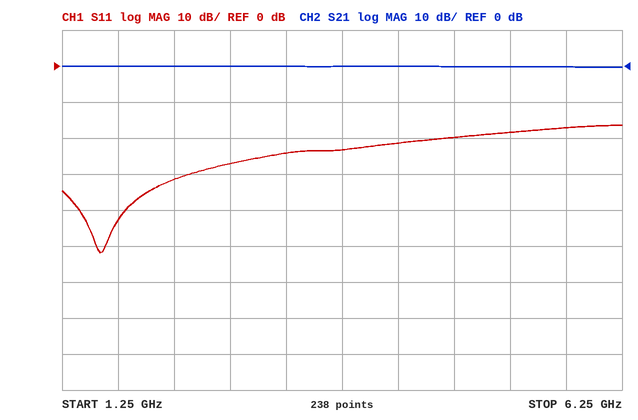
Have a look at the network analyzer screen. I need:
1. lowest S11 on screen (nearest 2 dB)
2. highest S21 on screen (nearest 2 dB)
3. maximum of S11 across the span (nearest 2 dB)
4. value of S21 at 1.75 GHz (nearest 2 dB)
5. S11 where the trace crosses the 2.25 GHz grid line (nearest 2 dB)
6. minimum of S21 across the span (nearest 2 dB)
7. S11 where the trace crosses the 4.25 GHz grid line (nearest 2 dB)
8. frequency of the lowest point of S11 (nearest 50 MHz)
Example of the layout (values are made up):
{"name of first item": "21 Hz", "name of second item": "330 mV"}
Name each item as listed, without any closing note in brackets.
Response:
{"lowest S11 on screen": "-52 dB", "highest S21 on screen": "0 dB", "maximum of S11 across the span": "-16 dB", "value of S21 at 1.75 GHz": "0 dB", "S11 where the trace crosses the 2.25 GHz grid line": "-32 dB", "minimum of S21 across the span": "0 dB", "S11 where the trace crosses the 4.25 GHz grid line": "-22 dB", "frequency of the lowest point of S11": "1.60 GHz"}
